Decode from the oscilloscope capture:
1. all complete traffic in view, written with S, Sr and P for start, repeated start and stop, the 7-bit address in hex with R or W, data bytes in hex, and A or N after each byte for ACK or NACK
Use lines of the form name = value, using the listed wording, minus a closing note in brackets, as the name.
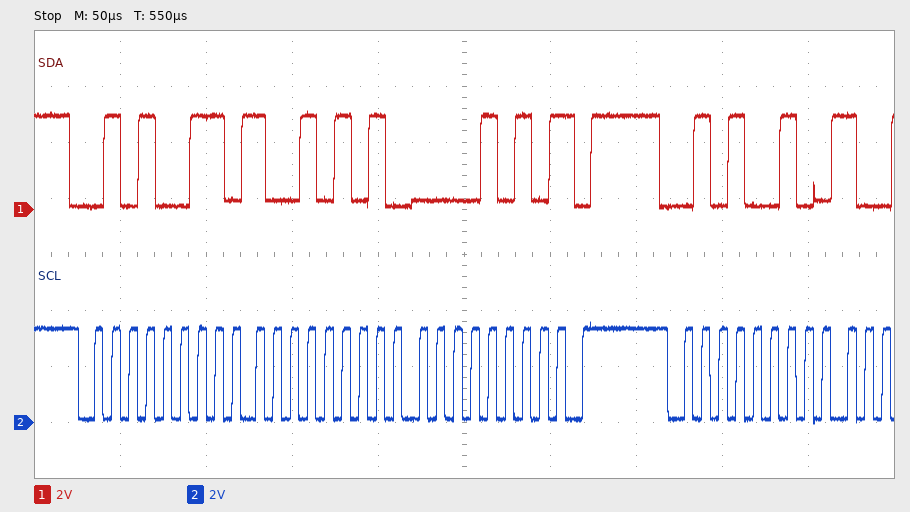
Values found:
all complete traffic in view, written with S, Sr and P for start, repeated start and stop, the 7-bit address in hex with R or W, data bytes in hex, and A or N after each byte for ACK or NACK = S 29R A 95 A 0A N P S 29W A
